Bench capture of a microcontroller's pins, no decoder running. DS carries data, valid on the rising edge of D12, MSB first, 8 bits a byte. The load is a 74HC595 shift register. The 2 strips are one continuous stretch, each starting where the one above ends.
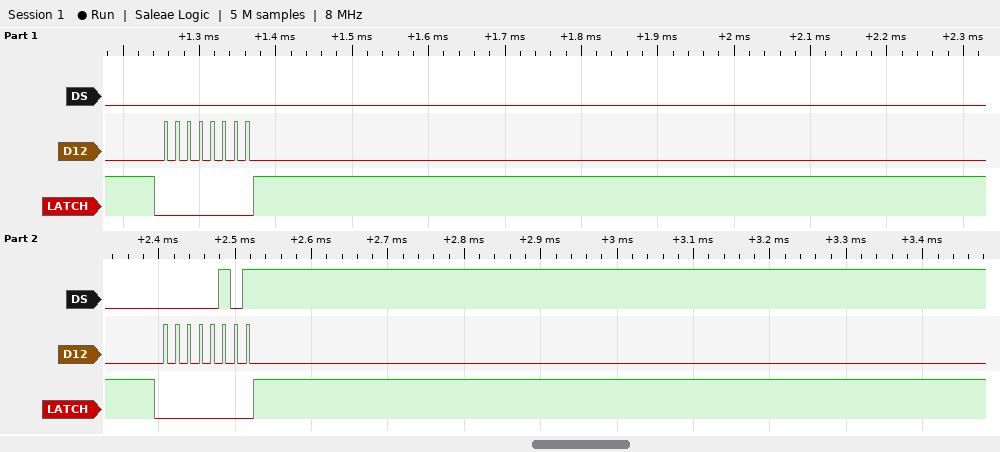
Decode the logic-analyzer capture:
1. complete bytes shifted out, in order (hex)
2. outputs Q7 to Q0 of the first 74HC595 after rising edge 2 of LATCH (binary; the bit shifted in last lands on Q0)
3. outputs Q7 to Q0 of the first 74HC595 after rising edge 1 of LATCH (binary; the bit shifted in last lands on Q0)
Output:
0x00 0x05
00000101
00000000
